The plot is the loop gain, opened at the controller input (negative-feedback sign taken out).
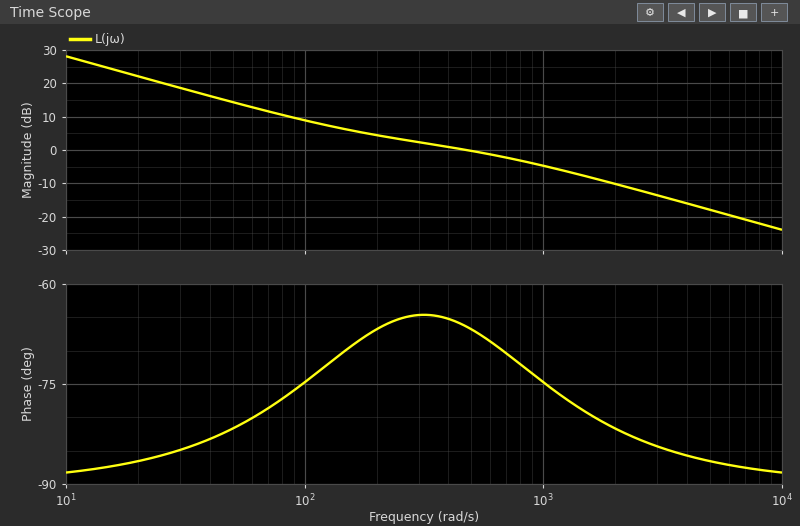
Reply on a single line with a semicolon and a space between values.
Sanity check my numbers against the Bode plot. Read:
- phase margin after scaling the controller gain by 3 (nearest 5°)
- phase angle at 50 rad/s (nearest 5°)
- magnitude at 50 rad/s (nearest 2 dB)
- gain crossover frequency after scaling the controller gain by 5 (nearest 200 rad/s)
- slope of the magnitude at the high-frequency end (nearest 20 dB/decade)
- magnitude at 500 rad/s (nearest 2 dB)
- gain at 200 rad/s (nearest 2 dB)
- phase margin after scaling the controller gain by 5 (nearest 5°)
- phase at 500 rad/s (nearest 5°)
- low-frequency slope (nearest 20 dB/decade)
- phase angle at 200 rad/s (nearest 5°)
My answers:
100°; -80°; 14 dB; 3200 rad/s; -20 dB/decade; 0 dB; 4 dB; 95°; -65°; -20 dB/decade; -65°
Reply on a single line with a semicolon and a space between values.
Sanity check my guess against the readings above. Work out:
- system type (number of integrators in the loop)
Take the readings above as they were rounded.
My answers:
1
